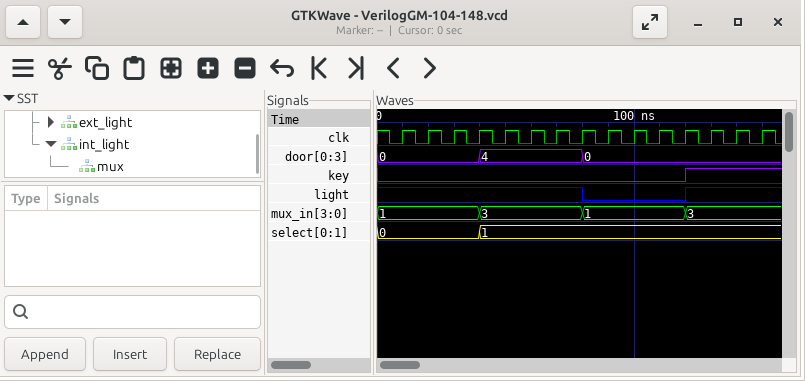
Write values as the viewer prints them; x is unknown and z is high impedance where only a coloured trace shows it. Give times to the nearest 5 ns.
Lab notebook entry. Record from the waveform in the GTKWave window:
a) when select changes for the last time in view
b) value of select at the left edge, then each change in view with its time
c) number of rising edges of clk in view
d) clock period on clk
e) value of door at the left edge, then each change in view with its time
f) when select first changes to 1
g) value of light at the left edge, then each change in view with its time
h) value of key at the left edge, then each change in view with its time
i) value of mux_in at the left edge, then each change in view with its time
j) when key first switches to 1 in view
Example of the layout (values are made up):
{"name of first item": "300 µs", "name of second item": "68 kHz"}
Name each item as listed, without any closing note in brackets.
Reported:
{"when select changes for the last time in view": "40 ns", "value of select at the left edge, then each change in view with its time": "0, 1 at 40 ns", "number of rising edges of clk in view": "15", "clock period on clk": "10 ns", "value of door at the left edge, then each change in view with its time": "0, 4 at 40 ns, 0 at 80 ns", "when select first changes to 1": "40 ns", "value of light at the left edge, then each change in view with its time": "1, 0 at 80 ns, 1 at 120 ns", "value of key at the left edge, then each change in view with its time": "0, 1 at 120 ns", "value of mux_in at the left edge, then each change in view with its time": "1, 3 at 40 ns, 1 at 80 ns, 3 at 120 ns", "when key first switches to 1 in view": "120 ns"}
